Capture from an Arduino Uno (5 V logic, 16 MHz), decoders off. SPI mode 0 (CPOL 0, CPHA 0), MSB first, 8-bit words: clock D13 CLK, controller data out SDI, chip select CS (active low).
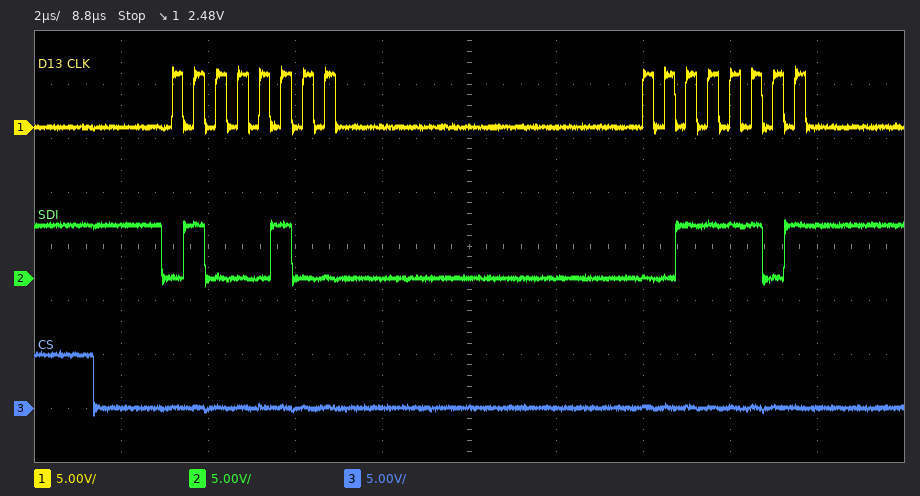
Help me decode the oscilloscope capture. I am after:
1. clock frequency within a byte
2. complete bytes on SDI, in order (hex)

2 MHz
0x44 0x3D
